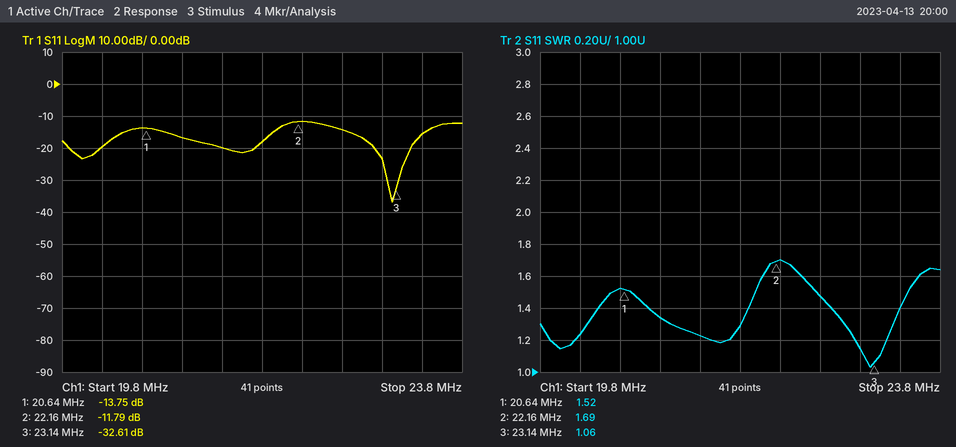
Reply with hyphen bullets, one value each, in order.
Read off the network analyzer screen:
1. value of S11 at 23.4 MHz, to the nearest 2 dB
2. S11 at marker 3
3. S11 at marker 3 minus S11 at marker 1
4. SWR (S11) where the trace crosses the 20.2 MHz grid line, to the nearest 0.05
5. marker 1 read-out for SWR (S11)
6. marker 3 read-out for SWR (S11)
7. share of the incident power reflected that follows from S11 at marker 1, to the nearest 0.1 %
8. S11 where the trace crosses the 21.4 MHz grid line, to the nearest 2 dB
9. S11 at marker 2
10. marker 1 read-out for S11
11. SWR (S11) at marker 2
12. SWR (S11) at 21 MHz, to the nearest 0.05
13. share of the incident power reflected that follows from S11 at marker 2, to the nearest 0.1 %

- -16 dB
- -32.61 dB
- -18.86 dB
- 1.25
- 1.52
- 1.06
- 4.2 %
- -20 dB
- -11.79 dB
- -13.75 dB
- 1.69
- 1.35
- 6.6 %
